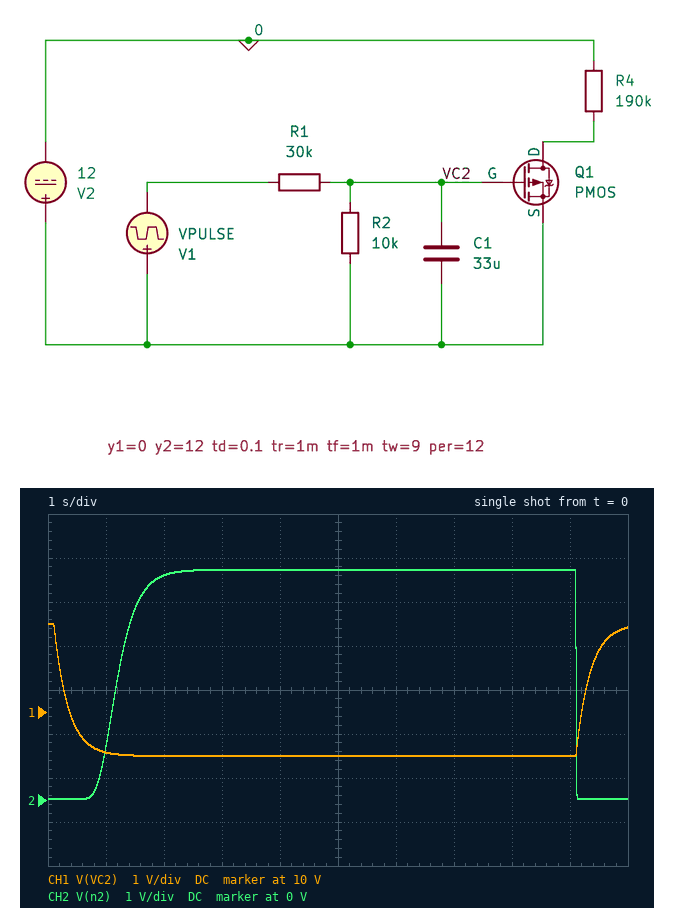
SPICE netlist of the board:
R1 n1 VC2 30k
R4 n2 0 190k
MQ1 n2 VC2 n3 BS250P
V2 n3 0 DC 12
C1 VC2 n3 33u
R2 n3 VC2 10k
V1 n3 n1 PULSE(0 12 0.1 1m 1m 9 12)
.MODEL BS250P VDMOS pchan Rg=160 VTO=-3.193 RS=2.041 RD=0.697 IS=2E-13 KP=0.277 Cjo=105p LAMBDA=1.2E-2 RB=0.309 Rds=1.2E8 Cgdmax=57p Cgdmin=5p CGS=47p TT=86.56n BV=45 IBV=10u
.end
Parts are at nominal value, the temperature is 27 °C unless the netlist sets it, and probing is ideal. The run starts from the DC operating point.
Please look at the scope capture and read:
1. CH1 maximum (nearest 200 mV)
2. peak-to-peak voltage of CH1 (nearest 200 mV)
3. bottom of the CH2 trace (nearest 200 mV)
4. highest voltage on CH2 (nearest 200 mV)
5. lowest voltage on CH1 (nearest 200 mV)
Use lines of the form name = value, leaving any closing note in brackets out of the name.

CH1 maximum = 12.0 V
peak-to-peak voltage of CH1 = 3.0 V
bottom of the CH2 trace = 0 V
highest voltage on CH2 = 5.2 V
lowest voltage on CH1 = 9.0 V
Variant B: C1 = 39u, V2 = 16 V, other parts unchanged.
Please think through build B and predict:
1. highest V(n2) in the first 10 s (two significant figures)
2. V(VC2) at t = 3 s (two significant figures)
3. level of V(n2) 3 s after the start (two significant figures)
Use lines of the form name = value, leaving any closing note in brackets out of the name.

highest V(n2) in the first 10 s = 5.5 V
V(VC2) at t = 3 s = 13 V
level of V(n2) 3 s after the start = 5.4 V
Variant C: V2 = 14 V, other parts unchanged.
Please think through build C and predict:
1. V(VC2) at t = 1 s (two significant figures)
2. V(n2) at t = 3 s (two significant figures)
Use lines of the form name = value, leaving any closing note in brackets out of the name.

V(VC2) at t = 1 s = 11 V
V(n2) at t = 3 s = 5.3 V
